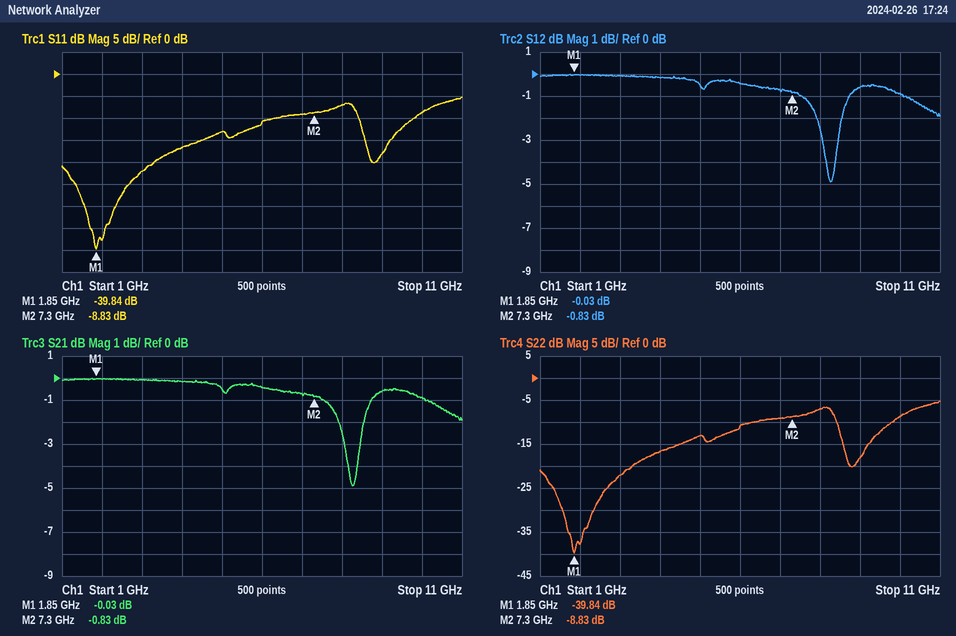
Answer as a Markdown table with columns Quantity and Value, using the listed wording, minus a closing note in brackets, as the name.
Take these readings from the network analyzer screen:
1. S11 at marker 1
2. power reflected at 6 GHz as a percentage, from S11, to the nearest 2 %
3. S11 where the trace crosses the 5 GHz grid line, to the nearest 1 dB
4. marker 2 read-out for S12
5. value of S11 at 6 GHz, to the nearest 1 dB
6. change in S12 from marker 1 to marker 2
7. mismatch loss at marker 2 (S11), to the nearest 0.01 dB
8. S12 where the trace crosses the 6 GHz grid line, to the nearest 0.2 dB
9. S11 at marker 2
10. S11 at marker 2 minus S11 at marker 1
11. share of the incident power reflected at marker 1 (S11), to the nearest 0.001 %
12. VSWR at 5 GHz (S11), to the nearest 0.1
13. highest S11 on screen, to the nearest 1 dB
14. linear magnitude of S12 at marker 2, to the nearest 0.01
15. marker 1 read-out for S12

| Quantity | Value |
|---|---|
| S11 at marker 1 | -39.84 dB |
| power reflected at 6 GHz as a percentage, from S11, to the nearest 2 % | 8 % |
| S11 where the trace crosses the 5 GHz grid line, to the nearest 1 dB | -13 dB |
| marker 2 read-out for S12 | -0.83 dB |
| value of S11 at 6 GHz, to the nearest 1 dB | -11 dB |
| change in S12 from marker 1 to marker 2 | -0.80 dB |
| mismatch loss at marker 2 (S11), to the nearest 0.01 dB | 0.61 dB |
| S12 where the trace crosses the 6 GHz grid line, to the nearest 0.2 dB | -0.4 dB |
| S11 at marker 2 | -8.83 dB |
| S11 at marker 2 minus S11 at marker 1 | 31.01 dB |
| share of the incident power reflected at marker 1 (S11), to the nearest 0.001 % | 0.010 % |
| VSWR at 5 GHz (S11), to the nearest 0.1 | 1.6 |
| highest S11 on screen, to the nearest 1 dB | -5 dB |
| linear magnitude of S12 at marker 2, to the nearest 0.01 | 0.91 |
| marker 1 read-out for S12 | -0.03 dB |
